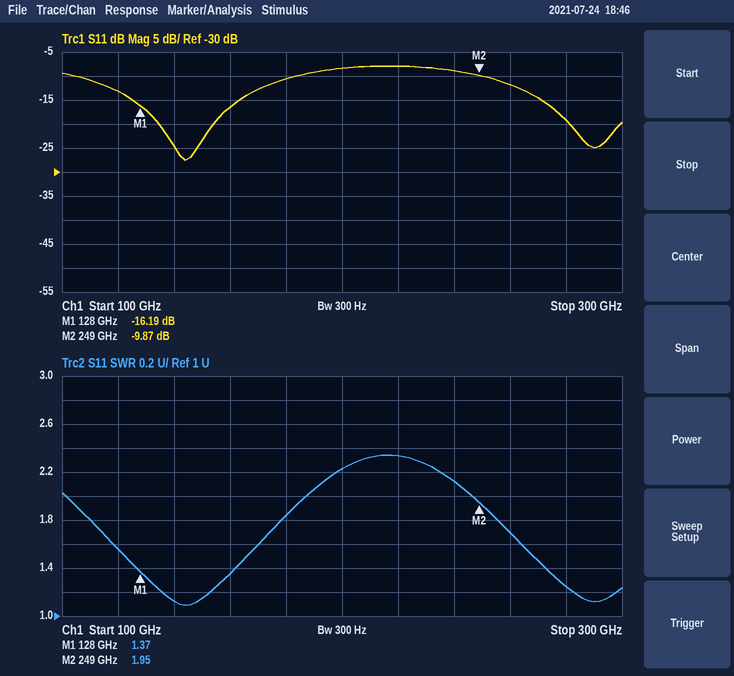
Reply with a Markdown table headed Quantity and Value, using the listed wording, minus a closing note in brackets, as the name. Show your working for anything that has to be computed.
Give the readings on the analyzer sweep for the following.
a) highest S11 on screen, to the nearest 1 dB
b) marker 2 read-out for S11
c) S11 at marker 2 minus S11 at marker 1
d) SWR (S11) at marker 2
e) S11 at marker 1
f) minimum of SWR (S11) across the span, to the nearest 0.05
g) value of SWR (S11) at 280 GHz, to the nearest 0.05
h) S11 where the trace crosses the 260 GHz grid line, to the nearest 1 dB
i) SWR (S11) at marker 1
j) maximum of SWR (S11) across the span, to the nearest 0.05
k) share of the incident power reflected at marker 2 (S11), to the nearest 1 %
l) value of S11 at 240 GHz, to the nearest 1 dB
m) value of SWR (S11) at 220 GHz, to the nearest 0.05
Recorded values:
| Quantity | Value |
|---|---|
| highest S11 on screen, to the nearest 1 dB | -8 dB |
| marker 2 read-out for S11 | -9.87 dB |
| S11 at marker 2 minus S11 at marker 1 | -9.87 − (-16.19) = 6.32 dB |
| SWR (S11) at marker 2 | 1.95 |
| S11 at marker 1 | -16.19 dB |
| minimum of SWR (S11) across the span, to the nearest 0.05 | 1.10 |
| value of SWR (S11) at 280 GHz, to the nearest 0.05 | 1.25 |
| S11 where the trace crosses the 260 GHz grid line, to the nearest 1 dB | -12 dB |
| SWR (S11) at marker 1 | 1.37 |
| maximum of SWR (S11) across the span, to the nearest 0.05 | 2.35 |
| share of the incident power reflected at marker 2 (S11), to the nearest 1 % | 10^(-9.87/10) ≈ 10 % |
| value of S11 at 240 GHz, to the nearest 1 dB | -9 dB |
| value of SWR (S11) at 220 GHz, to the nearest 0.05 | 2.35 |
